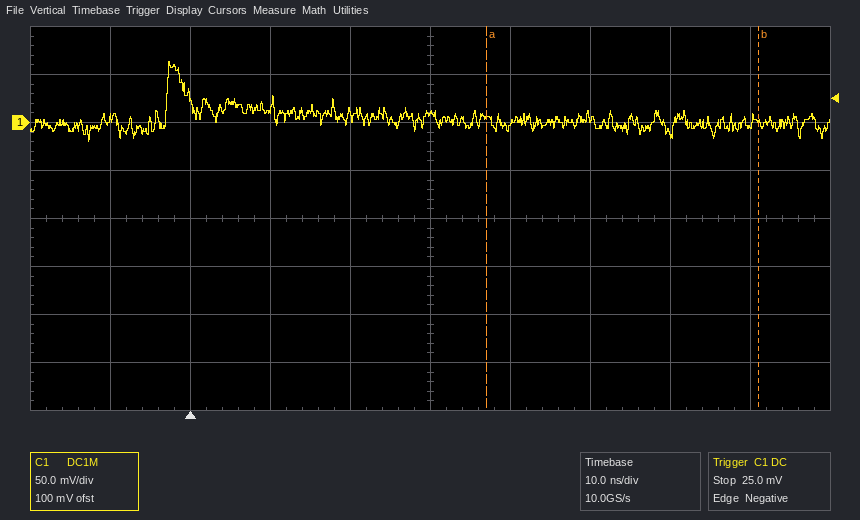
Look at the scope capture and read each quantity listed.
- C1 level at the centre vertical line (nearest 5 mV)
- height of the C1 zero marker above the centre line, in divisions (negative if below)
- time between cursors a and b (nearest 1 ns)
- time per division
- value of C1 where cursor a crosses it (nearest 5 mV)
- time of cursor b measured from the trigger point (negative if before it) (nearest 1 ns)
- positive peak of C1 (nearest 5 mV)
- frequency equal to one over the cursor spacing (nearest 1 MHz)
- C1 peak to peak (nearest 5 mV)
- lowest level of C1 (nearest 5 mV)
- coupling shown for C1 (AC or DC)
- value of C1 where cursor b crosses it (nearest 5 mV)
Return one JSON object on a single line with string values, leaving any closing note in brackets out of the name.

{"C1 level at the centre vertical line": "10 mV", "height of the C1 zero marker above the centre line, in divisions": "+2.0 div", "time between cursors a and b": "34 ns", "time per division": "10 ns", "value of C1 where cursor a crosses it": "5 mV", "time of cursor b measured from the trigger point (negative if before it)": "+71 ns", "positive peak of C1": "65 mV", "frequency equal to one over the cursor spacing": "29 MHz", "C1 peak to peak": "85 mV", "lowest level of C1": "-20 mV", "coupling shown for C1": "DC", "value of C1 where cursor b crosses it": "0 mV"}
